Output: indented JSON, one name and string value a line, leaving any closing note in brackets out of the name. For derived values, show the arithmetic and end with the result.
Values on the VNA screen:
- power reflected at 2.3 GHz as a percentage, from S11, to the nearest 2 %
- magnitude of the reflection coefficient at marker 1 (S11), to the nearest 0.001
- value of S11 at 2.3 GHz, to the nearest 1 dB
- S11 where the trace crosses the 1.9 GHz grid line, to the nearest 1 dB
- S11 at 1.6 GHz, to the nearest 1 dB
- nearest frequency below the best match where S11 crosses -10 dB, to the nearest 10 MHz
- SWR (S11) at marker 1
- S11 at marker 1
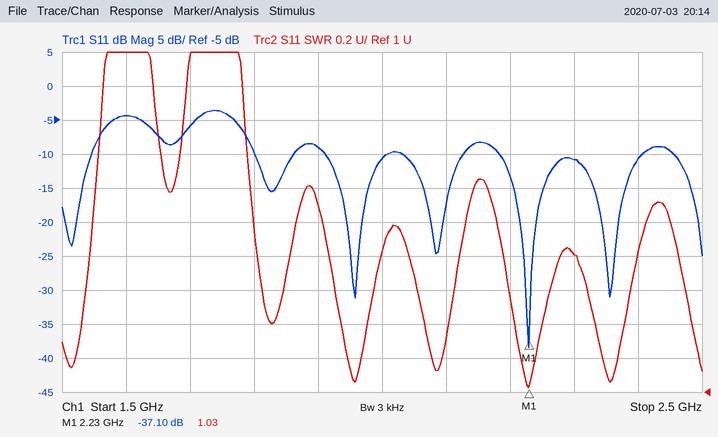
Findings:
{
  "power reflected at 2.3 GHz as a percentage, from S11, to the nearest 2 %": "10^(-11/10) ≈ 8 %",
  "magnitude of the reflection coefficient at marker 1 (S11), to the nearest 0.001": "10^(-37.1/20) ≈ 0.014",
  "value of S11 at 2.3 GHz, to the nearest 1 dB": "-11 dB",
  "S11 where the trace crosses the 1.9 GHz grid line, to the nearest 1 dB": "-9 dB",
  "S11 at 1.6 GHz, to the nearest 1 dB": "-4 dB",
  "nearest frequency below the best match where S11 crosses -10 dB, to the nearest 10 MHz": "2.18 GHz",
  "SWR (S11) at marker 1": "1.03",
  "S11 at marker 1": "-37.10 dB"
}
